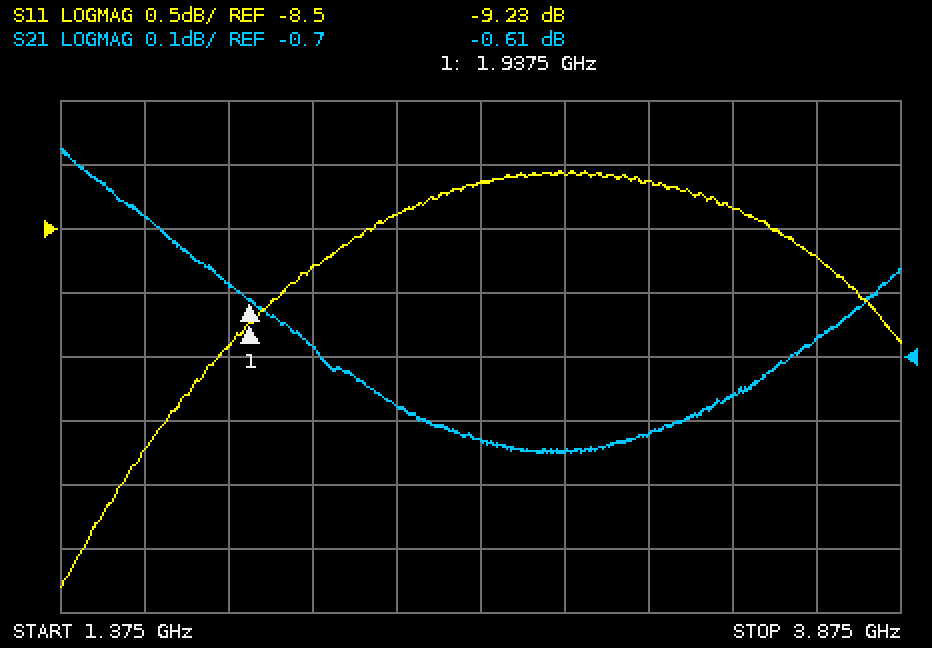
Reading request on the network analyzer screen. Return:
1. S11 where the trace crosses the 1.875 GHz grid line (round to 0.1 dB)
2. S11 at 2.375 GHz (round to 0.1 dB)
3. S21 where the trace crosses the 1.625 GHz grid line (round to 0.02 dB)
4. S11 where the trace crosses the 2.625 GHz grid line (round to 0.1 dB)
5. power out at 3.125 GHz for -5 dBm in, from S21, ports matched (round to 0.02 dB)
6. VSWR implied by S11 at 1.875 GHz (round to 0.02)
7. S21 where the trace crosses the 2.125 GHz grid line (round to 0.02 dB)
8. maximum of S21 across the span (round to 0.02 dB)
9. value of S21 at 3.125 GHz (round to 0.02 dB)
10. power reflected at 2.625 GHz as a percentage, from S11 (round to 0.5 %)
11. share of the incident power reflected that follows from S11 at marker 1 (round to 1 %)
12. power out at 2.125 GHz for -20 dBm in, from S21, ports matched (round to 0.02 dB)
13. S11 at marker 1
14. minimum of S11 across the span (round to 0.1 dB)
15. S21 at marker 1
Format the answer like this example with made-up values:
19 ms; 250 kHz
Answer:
-9.4 dB; -8.4 dB; -0.48 dB; -8.1 dB; -5.82 dBm; 2.02; -0.68 dB; -0.38 dB; -0.82 dB; 15.5 %; 12 %; -20.68 dBm; -9.23 dB; -11.3 dB; -0.61 dB
